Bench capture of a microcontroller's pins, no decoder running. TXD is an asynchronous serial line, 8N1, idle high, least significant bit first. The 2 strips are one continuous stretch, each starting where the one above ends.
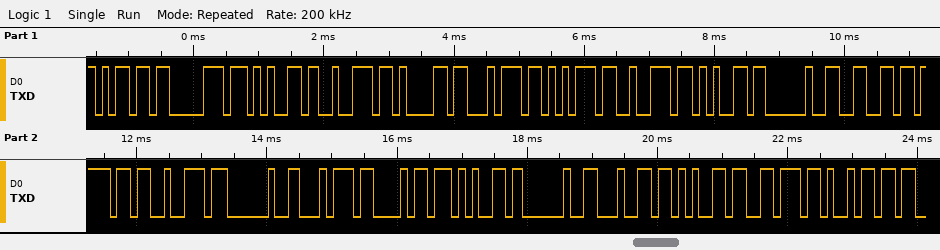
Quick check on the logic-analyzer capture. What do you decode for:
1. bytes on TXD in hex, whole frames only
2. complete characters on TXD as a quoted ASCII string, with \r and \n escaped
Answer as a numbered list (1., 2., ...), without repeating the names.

1. 6D 70 65 72 61 74 75 72 65 20 66 6F 72 20 74 68 65 20 64 65 76 69
2. "mperature for the devi"
